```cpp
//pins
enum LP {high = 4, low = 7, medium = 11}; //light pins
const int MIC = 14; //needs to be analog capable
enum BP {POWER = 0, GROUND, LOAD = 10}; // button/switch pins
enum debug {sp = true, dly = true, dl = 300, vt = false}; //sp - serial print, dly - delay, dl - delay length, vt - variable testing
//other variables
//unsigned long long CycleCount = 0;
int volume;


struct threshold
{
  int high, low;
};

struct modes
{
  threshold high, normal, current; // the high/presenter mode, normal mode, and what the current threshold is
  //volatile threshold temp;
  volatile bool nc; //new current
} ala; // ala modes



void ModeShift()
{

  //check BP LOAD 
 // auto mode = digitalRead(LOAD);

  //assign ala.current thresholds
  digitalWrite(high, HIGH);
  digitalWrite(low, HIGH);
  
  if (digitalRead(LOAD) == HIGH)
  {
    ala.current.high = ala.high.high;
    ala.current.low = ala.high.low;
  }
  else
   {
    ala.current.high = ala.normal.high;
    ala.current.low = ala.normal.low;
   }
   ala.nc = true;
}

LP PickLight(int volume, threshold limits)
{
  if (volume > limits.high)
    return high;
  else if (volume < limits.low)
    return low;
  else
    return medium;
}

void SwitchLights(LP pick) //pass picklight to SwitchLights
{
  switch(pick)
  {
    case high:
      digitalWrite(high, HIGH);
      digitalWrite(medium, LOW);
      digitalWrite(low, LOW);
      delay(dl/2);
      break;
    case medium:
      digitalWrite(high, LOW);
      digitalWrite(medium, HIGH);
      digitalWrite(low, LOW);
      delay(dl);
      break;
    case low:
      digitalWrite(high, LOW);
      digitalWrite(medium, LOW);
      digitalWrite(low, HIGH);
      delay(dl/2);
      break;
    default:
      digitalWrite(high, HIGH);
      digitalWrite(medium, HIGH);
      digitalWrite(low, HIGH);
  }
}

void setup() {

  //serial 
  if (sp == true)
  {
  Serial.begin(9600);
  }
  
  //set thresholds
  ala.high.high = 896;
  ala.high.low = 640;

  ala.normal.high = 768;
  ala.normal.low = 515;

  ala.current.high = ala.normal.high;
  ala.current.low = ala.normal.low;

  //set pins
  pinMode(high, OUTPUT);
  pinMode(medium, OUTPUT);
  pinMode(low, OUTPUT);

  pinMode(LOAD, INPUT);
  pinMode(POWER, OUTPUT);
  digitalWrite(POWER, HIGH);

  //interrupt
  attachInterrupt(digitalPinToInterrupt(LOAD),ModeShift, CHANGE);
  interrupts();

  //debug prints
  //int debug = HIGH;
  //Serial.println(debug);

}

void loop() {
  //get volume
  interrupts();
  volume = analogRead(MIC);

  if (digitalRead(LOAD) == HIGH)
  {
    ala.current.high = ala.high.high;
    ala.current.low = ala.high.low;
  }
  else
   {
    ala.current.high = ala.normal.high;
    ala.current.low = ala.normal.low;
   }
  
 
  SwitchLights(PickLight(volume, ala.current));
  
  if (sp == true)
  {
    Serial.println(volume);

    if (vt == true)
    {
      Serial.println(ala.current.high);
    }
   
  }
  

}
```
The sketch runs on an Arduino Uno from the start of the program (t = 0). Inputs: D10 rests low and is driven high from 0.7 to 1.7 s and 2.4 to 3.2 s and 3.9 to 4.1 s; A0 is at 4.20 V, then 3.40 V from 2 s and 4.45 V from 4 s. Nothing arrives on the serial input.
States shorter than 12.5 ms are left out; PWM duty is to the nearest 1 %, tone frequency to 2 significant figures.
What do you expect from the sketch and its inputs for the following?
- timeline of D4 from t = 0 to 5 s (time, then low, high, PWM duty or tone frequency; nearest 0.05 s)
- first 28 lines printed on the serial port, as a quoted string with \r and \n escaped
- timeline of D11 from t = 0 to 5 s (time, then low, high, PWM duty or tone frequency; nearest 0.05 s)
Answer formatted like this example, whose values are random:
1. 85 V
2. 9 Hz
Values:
1. 0 s high; 0.75 s low; 1.95 s high; 2.1 s low; 4.2 s high
2. "860\r\n860\r\n860\r\n860\r\n860\r\n860\r\n860\r\n860\r\n860\r\n860\r\n696\r\n696\r\n696\r\n696\r\n696\r\n696\r\n696\r\n911\r\n911\r\n911\r\n911\r\n911\r\n911\r\n911\r\n911\r\n911\r\n911\r\n911\r\n"
3. 0 s low; 0.75 s high; 1.95 s low; 2.1 s high; 4.2 s low
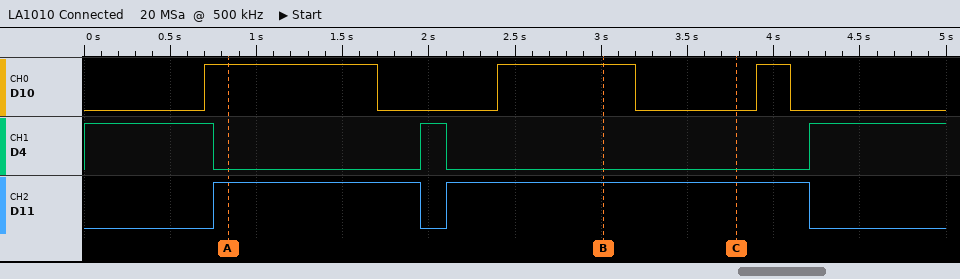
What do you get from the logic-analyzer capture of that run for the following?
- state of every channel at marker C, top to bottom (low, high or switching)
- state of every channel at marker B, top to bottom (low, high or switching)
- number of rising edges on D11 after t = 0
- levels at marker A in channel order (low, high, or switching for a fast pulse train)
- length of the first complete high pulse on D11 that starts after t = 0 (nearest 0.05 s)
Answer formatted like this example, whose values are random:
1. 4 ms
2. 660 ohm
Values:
1. D10 low, D4 low, D11 high
2. D10 high, D4 low, D11 high
3. 2
4. D10 high, D4 low, D11 high
5. 1.20 s
